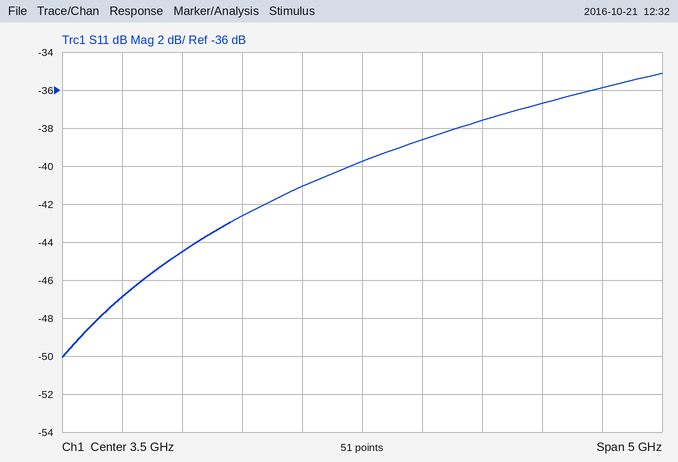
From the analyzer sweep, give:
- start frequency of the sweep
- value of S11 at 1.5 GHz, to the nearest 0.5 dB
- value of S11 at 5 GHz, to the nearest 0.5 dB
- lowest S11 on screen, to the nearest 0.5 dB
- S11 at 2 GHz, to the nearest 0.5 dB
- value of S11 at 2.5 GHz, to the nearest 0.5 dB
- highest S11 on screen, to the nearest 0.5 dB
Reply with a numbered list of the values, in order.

1. 1 GHz
2. -47.0 dB
3. -36.5 dB
4. -50.0 dB
5. -44.5 dB
6. -42.5 dB
7. -35.0 dB
